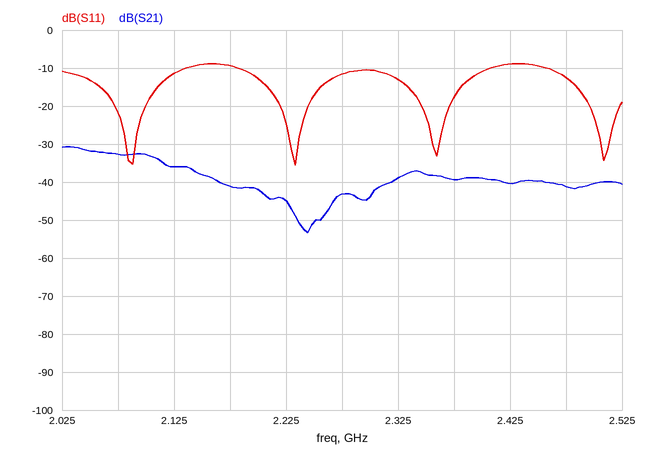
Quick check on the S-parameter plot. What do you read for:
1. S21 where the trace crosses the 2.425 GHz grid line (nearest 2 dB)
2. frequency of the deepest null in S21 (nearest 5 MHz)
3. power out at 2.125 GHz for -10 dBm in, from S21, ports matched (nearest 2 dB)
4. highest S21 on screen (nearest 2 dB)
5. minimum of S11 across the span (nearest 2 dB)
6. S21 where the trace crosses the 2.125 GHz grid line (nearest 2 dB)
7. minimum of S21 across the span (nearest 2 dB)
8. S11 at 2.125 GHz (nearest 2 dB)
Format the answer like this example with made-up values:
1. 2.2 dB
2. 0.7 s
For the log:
1. -40 dB
2. 2.245 GHz
3. -46 dBm
4. -30 dB
5. -36 dB
6. -36 dB
7. -54 dB
8. -12 dB
